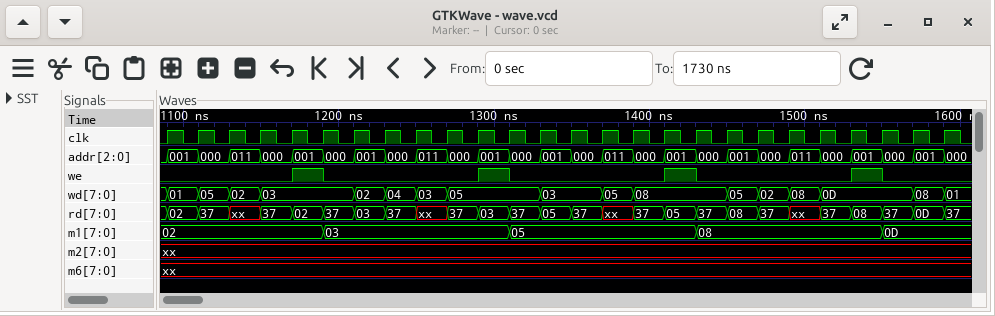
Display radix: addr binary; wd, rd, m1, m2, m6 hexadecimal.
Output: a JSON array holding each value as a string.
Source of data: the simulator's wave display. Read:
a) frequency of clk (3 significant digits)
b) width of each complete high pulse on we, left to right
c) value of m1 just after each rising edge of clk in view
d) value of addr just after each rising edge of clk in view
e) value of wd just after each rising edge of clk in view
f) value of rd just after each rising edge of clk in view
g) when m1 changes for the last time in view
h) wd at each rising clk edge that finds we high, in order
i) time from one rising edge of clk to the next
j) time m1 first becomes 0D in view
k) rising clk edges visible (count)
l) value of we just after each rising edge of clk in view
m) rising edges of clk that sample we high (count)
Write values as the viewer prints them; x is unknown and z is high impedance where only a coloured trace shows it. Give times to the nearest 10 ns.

["50.0 MHz", "20 ns, 20 ns, 20 ns, 20 ns", "02, 02, 02, 02, 02, 03, 03, 03, 03, 03, 03, 05, 05, 05, 05, 05, 05, 08, 08, 08, 08, 08, 08, 0D, 0D, 0D", "001, 000, 011, 000, 001, 000, 001, 000, 011, 000, 001, 000, 001, 000, 011, 000, 001, 000, 001, 000, 011, 000, 001, 000, 001, 000", "01, 05, 02, 03, 03, 03, 02, 04, 03, 05, 05, 05, 03, 03, 05, 08, 08, 08, 05, 02, 08, 0D, 0D, 0D, 08, 01", "02, 37, xx, 37, 02, 37, 03, 37, xx, 37, 03, 37, 05, 37, xx, 37, 05, 37, 08, 37, xx, 37, 08, 37, 0D, 37", "1550 ns", "03, 05, 08, 0D", "20 ns", "1550 ns", "26", "0 0 0 0 1 0 0 0 0 0 1 0 0 0 0 0 1 0 0 0 0 0 1 0 0 0", "4"]
